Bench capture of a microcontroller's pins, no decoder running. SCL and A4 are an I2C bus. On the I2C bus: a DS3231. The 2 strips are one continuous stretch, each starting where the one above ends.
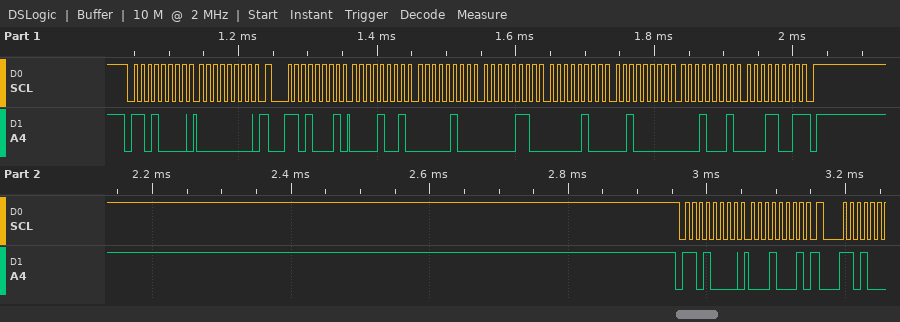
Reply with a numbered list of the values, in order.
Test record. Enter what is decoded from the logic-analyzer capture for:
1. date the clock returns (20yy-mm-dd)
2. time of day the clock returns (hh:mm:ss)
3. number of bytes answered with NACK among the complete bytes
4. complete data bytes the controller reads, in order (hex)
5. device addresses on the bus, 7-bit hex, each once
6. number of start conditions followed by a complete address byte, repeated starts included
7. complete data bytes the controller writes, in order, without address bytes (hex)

1. 2019-11-20
2. 06:04:09
3. 1
4. 09 04 06 04 20 11 19
5. 0x68
6. 3
7. 00 11
